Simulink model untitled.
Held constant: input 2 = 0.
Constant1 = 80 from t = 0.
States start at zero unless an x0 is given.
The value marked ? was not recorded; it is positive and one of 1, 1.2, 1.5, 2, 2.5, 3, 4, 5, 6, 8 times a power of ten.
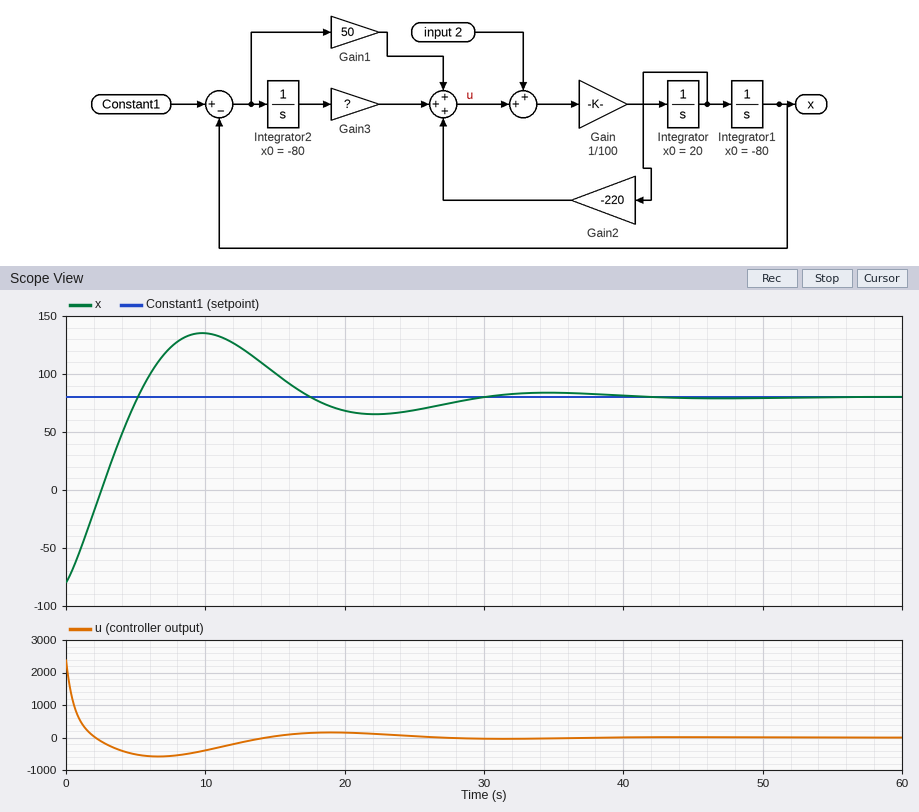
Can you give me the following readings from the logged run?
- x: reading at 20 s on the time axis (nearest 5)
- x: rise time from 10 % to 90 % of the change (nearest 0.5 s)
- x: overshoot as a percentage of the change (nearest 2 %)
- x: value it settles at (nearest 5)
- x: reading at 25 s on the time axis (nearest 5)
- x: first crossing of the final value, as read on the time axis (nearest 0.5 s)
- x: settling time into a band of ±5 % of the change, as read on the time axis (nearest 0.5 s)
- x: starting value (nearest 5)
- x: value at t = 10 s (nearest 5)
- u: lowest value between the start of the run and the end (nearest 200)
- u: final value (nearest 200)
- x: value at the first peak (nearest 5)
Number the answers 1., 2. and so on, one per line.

1. 70
2. 4.0 s
3. 34 %
4. 80
5. 70
6. 5.0 s
7. 26.5 s
8. -80
9. 135
10. -600
11. 0
12. 135
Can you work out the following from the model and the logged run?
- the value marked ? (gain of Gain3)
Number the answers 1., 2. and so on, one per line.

1. 15
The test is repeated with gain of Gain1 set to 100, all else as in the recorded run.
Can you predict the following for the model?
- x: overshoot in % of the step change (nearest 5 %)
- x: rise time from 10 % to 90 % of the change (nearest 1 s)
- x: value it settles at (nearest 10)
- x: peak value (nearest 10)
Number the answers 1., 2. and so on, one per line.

1. 15 %
2. 3 s
3. 80
4. 100
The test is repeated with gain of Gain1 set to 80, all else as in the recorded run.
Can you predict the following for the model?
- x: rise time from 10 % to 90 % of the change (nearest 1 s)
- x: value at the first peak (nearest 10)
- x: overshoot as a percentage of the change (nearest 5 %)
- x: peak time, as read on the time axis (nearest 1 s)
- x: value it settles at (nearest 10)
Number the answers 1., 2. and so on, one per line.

1. 3 s
2. 110
3. 20 %
4. 8 s
5. 80
